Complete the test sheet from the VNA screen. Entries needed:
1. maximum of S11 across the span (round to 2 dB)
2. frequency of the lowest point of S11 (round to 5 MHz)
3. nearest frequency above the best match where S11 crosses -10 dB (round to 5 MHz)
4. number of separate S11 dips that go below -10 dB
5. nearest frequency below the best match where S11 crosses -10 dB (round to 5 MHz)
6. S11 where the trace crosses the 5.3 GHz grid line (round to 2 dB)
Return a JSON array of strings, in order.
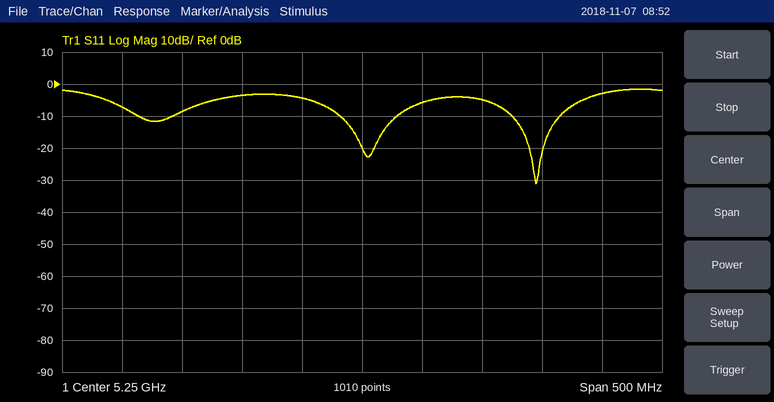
["-2 dB", "5.395 GHz", "5.415 GHz", "3", "5.375 GHz", "-6 dB"]
